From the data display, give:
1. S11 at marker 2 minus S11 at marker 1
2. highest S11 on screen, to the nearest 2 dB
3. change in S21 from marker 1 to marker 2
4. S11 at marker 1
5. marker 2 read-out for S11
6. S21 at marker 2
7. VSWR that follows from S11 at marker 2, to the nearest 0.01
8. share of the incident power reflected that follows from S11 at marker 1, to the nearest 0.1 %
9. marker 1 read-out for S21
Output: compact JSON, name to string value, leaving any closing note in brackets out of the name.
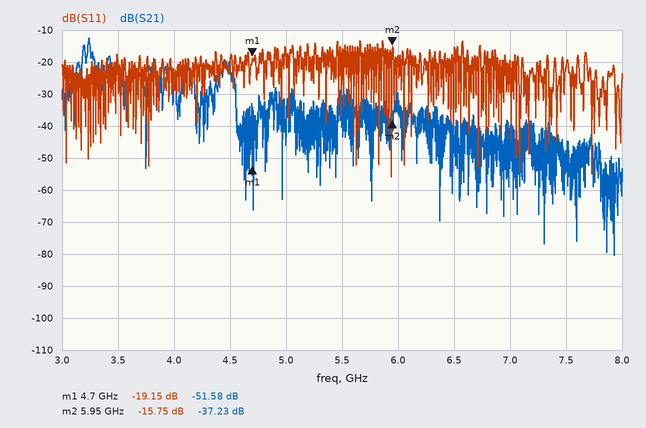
{"S11 at marker 2 minus S11 at marker 1": "3.40 dB", "highest S11 on screen, to the nearest 2 dB": "-14 dB", "change in S21 from marker 1 to marker 2": "14.35 dB", "S11 at marker 1": "-19.15 dB", "marker 2 read-out for S11": "-15.75 dB", "S21 at marker 2": "-37.23 dB", "VSWR that follows from S11 at marker 2, to the nearest 0.01": "1.39", "share of the incident power reflected that follows from S11 at marker 1, to the nearest 0.1 %": "1.2 %", "marker 1 read-out for S21": "-51.58 dB"}
